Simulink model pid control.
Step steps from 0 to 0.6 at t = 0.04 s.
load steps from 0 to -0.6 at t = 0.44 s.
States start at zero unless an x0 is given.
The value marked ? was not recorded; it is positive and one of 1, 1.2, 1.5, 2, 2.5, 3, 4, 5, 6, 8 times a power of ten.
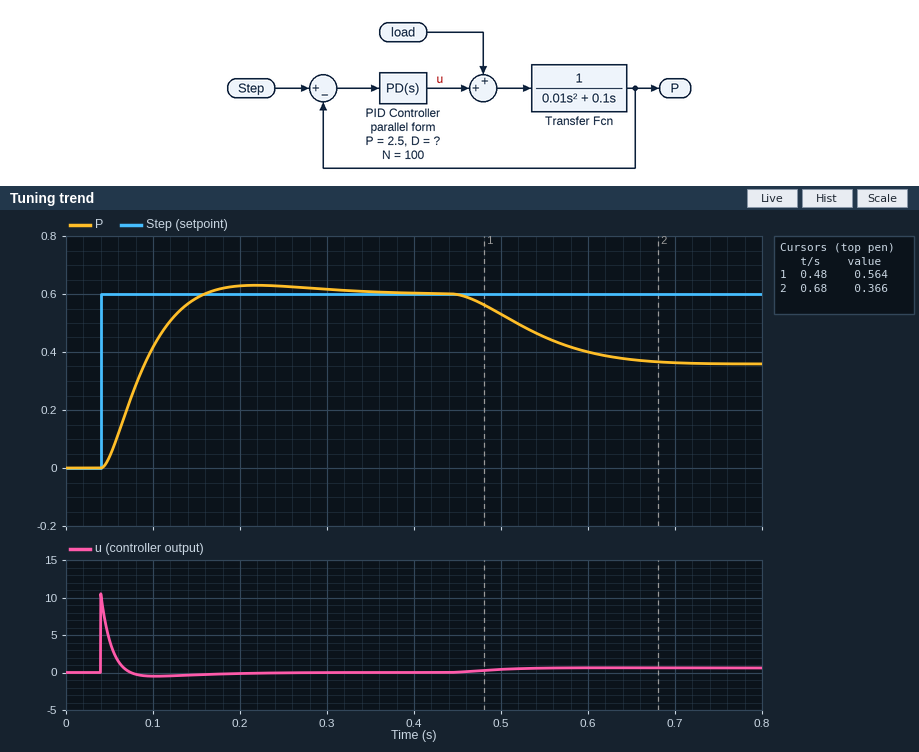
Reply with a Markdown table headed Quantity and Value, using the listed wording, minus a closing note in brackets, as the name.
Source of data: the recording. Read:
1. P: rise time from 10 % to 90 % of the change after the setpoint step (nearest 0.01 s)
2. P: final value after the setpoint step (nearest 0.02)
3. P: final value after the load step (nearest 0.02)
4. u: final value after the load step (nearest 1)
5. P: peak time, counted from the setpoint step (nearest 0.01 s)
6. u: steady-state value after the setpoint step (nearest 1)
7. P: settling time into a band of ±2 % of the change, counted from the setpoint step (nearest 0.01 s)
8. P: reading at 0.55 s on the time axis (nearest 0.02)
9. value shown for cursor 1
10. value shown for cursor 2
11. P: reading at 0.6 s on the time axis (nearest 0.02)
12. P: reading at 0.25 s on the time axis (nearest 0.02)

| Quantity | Value |
|---|---|
| P: rise time from 10 % to 90 % of the change after the setpoint step | 0.08 s |
| P: final value after the setpoint step | 0.60 |
| P: final value after the load step | 0.36 |
| u: final value after the load step | 1 |
| P: peak time, counted from the setpoint step | 0.18 s |
| u: steady-state value after the setpoint step | 0 |
| P: settling time into a band of ±2 % of the change, counted from the setpoint step | 0.28 s |
| P: reading at 0.55 s on the time axis | 0.46 |
| value shown for cursor 1 | 0.564 |
| value shown for cursor 2 | 0.366 |
| P: reading at 0.6 s on the time axis | 0.40 |
| P: reading at 0.25 s on the time axis | 0.62 |
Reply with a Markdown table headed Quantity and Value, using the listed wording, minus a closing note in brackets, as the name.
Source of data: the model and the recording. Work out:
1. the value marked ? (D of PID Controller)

| Quantity | Value |
|---|---|
| the value marked ? | 0.15 |
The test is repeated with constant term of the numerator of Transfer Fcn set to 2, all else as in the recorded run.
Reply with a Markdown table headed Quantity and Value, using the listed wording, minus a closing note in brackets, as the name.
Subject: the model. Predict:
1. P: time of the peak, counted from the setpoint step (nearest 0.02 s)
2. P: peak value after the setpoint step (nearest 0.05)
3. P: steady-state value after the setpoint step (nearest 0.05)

| Quantity | Value |
|---|---|
| P: time of the peak, counted from the setpoint step | 0.08 s |
| P: peak value after the setpoint step | 0.65 |
| P: steady-state value after the setpoint step | 0.60 |
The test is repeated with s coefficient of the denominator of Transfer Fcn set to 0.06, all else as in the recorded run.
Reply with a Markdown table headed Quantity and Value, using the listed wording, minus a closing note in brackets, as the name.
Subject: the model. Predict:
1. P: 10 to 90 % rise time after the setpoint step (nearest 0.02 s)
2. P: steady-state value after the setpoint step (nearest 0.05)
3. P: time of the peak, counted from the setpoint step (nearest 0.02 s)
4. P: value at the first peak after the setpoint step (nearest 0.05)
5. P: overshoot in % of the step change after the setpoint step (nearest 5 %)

| Quantity | Value |
|---|---|
| P: 10 to 90 % rise time after the setpoint step | 0.06 s |
| P: steady-state value after the setpoint step | 0.60 |
| P: time of the peak, counted from the setpoint step | 0.16 s |
| P: value at the first peak after the setpoint step | 0.70 |
| P: overshoot in % of the step change after the setpoint step | 15 % |
